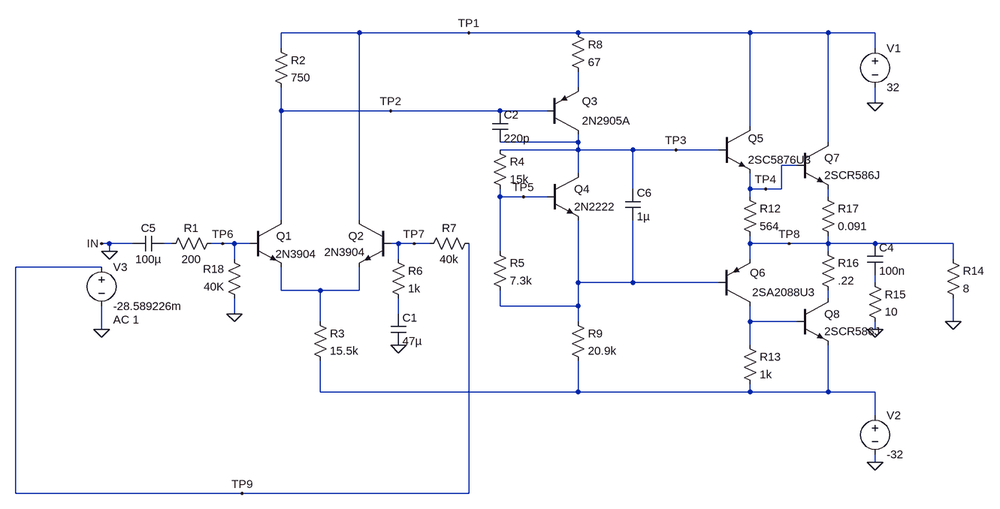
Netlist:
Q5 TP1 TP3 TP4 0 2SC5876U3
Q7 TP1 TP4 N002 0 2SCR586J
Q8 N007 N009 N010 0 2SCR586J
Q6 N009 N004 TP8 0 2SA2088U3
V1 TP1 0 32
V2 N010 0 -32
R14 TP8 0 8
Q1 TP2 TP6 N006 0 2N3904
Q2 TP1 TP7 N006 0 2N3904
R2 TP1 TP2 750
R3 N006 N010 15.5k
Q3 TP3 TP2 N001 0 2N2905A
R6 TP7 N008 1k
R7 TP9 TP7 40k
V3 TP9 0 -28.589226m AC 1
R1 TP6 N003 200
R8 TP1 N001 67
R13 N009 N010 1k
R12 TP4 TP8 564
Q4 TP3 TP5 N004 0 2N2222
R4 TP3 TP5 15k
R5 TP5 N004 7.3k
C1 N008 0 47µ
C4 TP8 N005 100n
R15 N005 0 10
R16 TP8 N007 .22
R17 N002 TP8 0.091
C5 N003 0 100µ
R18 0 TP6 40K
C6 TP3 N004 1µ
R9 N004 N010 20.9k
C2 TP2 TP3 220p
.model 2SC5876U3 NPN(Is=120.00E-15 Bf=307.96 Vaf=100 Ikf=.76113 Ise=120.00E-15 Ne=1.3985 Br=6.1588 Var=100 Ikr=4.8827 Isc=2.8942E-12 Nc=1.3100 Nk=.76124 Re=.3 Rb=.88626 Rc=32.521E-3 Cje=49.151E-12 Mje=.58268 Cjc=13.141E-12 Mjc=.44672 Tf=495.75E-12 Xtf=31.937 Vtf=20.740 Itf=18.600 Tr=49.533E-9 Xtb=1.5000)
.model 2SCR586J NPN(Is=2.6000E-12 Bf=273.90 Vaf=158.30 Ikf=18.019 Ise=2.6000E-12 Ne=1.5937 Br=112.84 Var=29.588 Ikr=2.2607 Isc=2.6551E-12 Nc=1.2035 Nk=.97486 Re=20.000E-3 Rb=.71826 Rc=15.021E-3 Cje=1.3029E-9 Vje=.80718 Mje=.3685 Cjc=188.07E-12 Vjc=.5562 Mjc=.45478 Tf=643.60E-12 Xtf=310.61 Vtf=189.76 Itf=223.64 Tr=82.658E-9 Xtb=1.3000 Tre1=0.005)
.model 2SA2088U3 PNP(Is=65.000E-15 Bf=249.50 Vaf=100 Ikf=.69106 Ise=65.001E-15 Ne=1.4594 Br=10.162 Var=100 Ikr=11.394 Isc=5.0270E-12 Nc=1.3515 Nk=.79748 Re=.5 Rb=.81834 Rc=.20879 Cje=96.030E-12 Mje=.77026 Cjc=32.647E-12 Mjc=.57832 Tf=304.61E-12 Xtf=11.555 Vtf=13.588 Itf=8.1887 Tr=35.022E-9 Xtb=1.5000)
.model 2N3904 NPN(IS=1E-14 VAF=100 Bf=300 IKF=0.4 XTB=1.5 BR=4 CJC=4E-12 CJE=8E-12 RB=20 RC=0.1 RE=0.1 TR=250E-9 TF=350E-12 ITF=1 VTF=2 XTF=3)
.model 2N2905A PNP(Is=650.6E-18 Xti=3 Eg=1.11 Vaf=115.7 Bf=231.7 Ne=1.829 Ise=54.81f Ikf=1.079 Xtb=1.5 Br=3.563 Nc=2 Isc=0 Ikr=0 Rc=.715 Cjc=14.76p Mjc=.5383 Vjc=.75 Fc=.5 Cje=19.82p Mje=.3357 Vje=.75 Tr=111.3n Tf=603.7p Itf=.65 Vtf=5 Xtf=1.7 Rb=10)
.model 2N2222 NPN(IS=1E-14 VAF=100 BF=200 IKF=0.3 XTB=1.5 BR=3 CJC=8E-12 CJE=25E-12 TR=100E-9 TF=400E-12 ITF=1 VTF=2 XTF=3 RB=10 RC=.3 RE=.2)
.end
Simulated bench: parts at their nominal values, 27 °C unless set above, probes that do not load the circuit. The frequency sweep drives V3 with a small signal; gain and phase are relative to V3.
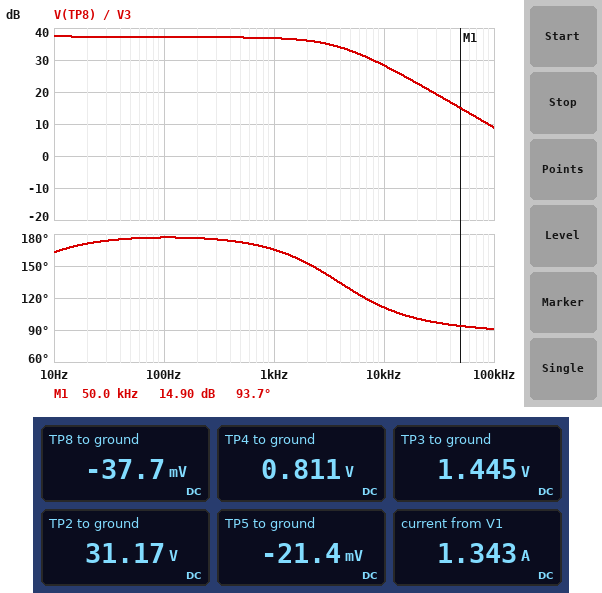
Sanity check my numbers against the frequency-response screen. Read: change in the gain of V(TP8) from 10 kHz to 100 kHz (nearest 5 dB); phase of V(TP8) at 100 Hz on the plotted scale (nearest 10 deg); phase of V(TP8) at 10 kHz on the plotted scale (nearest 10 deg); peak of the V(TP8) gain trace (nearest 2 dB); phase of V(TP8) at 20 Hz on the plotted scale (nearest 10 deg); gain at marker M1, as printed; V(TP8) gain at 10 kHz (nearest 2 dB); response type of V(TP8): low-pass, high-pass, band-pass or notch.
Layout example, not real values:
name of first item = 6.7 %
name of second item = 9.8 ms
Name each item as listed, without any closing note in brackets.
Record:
change in the gain of V(TP8) from 10 kHz to 100 kHz = -20 dB
phase of V(TP8) at 100 Hz on the plotted scale = 180 deg
phase of V(TP8) at 10 kHz on the plotted scale = 110 deg
peak of the V(TP8) gain trace = 38 dB
phase of V(TP8) at 20 Hz on the plotted scale = 170 deg
gain at marker M1, as printed = 14.90 dB
V(TP8) gain at 10 kHz = 28 dB
response type of V(TP8): low-pass, high-pass, band-pass or notch = low-pass
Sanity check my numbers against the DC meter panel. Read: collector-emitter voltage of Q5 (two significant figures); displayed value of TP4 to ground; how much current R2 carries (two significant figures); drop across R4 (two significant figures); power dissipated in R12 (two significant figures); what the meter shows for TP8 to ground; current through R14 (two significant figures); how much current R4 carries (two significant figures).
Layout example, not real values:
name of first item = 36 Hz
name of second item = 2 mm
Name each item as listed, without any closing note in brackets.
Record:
collector-emitter voltage of Q5 = 31 V
displayed value of TP4 to ground = 0.811 V
how much current R2 carries = 1.1 mA
drop across R4 = 1.5 V
power dissipated in R12 = 1.3 mW
what the meter shows for TP8 to ground = -37.7 mV
current through R14 = 4.7 mA
how much current R4 carries = 98 µA
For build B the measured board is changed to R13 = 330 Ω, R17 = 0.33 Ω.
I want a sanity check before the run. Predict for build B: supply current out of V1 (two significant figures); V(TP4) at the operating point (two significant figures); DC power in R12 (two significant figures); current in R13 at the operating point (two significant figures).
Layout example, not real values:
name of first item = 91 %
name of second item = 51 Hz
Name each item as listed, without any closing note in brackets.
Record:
supply current out of V1 = 580 mA
V(TP4) at the operating point = 900 mV
DC power in R12 = 1.4 mW
current in R13 at the operating point = 2.1 mA
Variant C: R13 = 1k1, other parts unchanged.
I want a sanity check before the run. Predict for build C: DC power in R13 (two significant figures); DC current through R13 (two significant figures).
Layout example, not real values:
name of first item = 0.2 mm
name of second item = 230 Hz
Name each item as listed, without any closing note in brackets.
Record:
DC power in R13 = 480 µW
DC current through R13 = 660 µA
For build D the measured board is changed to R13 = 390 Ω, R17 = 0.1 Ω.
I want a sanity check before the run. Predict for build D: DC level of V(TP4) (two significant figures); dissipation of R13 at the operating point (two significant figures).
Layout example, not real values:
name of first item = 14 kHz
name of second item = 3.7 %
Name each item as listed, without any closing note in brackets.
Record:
DC level of V(TP4) = 880 mV
dissipation of R13 at the operating point = 1.3 mW
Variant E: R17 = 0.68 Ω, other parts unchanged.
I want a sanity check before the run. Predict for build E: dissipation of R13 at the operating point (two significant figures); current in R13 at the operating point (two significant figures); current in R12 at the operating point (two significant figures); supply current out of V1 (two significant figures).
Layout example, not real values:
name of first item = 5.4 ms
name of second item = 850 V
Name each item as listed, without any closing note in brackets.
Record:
dissipation of R13 at the operating point = 450 µW
current in R13 at the operating point = 670 µA
current in R12 at the operating point = 1.6 mA
supply current out of V1 = 350 mA
